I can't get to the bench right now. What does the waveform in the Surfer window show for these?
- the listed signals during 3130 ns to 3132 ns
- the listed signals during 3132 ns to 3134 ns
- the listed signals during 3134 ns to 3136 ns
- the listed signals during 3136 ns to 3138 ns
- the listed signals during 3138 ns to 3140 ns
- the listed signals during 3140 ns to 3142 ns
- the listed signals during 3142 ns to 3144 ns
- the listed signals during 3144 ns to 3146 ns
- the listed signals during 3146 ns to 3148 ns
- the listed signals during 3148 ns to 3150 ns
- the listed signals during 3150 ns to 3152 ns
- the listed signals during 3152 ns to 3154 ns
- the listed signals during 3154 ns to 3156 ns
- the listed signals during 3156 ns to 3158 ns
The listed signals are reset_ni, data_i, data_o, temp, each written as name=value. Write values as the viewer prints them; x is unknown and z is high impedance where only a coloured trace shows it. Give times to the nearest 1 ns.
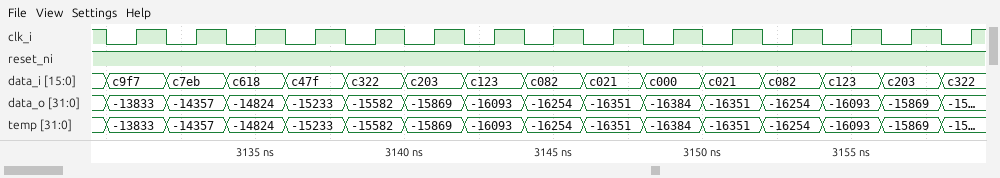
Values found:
reset_ni=1, data_i=c9f7, data_o=-13833, temp=-13833
reset_ni=1, data_i=c7eb, data_o=-14357, temp=-14357
reset_ni=1, data_i=c618, data_o=-14824, temp=-14824
reset_ni=1, data_i=c47f, data_o=-15233, temp=-15233
reset_ni=1, data_i=c322, data_o=-15582, temp=-15582
reset_ni=1, data_i=c203, data_o=-15869, temp=-15869
reset_ni=1, data_i=c123, data_o=-16093, temp=-16093
reset_ni=1, data_i=c082, data_o=-16254, temp=-16254
reset_ni=1, data_i=c021, data_o=-16351, temp=-16351
reset_ni=1, data_i=c000, data_o=-16384, temp=-16384
reset_ni=1, data_i=c021, data_o=-16351, temp=-16351
reset_ni=1, data_i=c082, data_o=-16254, temp=-16254
reset_ni=1, data_i=c123, data_o=-16093, temp=-16093
reset_ni=1, data_i=c203, data_o=-15869, temp=-15869
